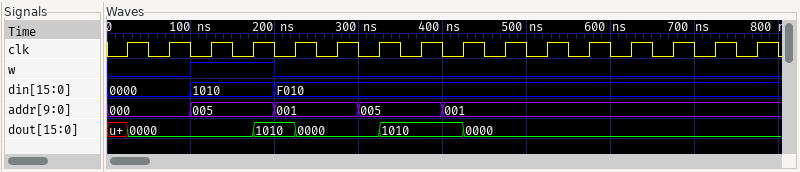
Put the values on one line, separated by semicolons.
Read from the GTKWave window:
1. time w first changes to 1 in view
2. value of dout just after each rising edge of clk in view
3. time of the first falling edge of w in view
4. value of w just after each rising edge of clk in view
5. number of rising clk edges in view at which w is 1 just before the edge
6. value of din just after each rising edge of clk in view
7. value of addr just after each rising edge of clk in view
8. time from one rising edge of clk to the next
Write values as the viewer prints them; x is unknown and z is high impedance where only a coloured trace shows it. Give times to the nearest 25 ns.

100 ns; 0000, 0000, 0000, 1010, 0000, 0000, 1010, 1010, 0000, 0000, 0000, 0000, 0000, 0000, 0000, 0000; 200 ns; 0 0 1 1 0 0 0 0 0 0 0 0 0 0 0 0; 2; 0000, 0000, 1010, 1010, F010, F010, F010, F010, F010, F010, F010, F010, F010, F010, F010, F010; 000, 000, 005, 005, 001, 001, 005, 005, 001, 001, 001, 001, 001, 001, 001, 001; 50 ns
